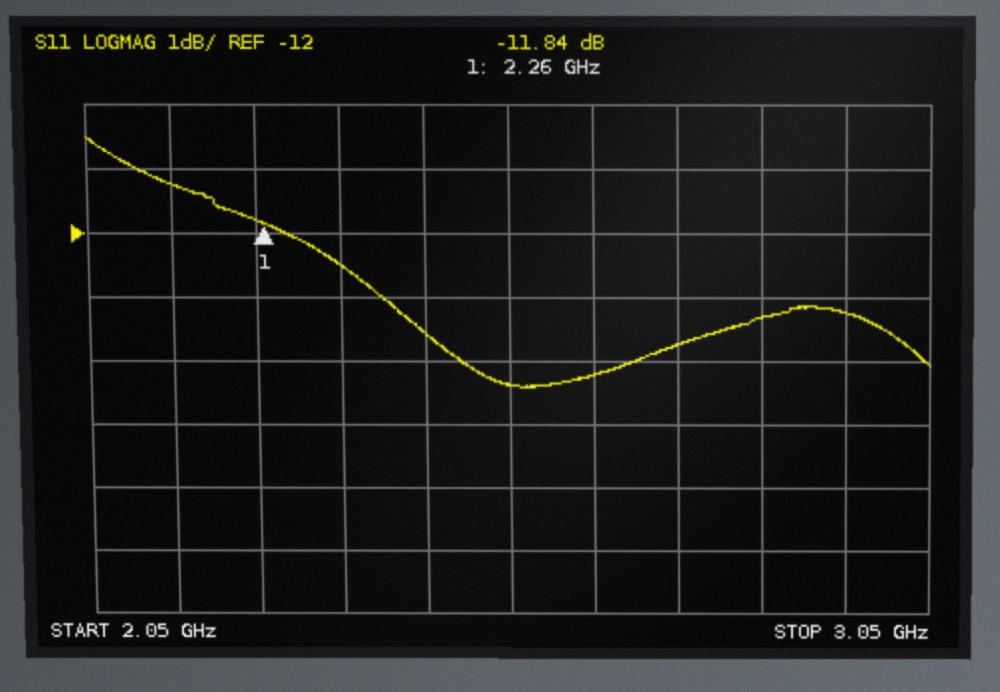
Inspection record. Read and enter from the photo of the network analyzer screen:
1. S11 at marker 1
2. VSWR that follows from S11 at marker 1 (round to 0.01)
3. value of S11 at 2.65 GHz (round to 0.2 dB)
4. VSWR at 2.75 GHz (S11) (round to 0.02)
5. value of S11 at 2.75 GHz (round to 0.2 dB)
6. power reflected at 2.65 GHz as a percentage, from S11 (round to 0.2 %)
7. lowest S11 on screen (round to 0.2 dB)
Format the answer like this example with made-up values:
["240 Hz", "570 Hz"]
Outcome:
["-11.84 dB", "1.69", "-14.2 dB", "1.52", "-13.8 dB", "3.8 %", "-14.4 dB"]
